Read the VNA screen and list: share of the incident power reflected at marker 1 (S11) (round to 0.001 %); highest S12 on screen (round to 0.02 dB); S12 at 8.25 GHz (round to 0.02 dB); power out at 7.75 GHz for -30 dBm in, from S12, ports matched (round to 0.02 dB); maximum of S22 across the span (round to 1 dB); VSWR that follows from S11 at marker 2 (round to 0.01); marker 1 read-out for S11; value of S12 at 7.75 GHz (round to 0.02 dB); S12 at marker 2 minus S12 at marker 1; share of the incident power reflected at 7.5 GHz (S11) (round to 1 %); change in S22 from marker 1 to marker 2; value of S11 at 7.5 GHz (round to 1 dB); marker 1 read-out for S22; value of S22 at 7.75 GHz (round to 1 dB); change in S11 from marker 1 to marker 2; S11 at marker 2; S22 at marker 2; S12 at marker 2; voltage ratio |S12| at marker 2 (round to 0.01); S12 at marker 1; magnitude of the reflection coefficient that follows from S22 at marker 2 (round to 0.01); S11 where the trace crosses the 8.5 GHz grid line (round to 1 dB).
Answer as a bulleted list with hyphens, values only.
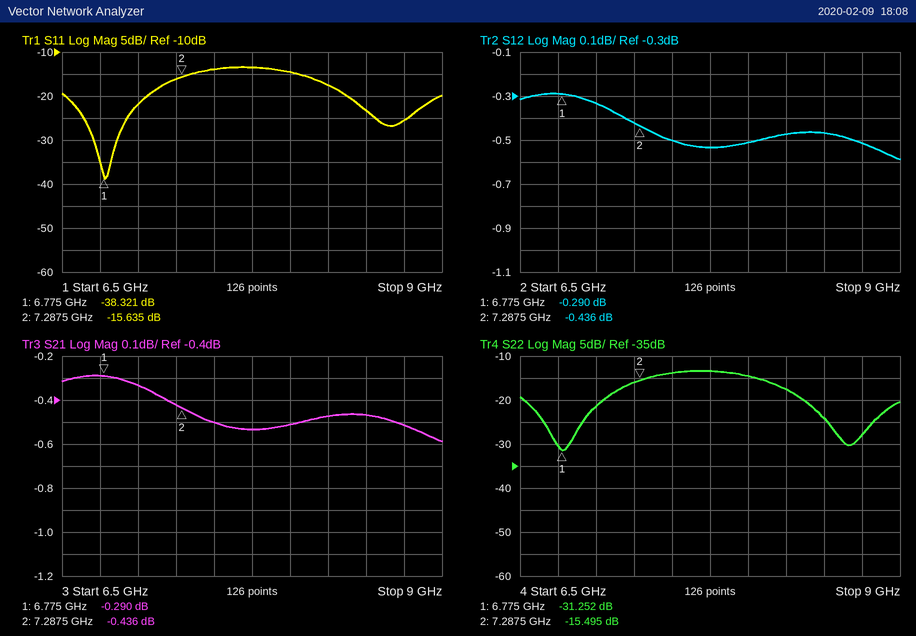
- 0.015 %
- -0.28 dB
- -0.48 dB
- -30.54 dBm
- -13 dB
- 1.40
- -38.321 dB
- -0.54 dB
- -0.146 dB
- 4 %
- 15.757 dB
- -14 dB
- -31.252 dB
- -13 dB
- 22.686 dB
- -15.635 dB
- -15.495 dB
- -0.436 dB
- 0.95
- -0.290 dB
- 0.17
- -23 dB
